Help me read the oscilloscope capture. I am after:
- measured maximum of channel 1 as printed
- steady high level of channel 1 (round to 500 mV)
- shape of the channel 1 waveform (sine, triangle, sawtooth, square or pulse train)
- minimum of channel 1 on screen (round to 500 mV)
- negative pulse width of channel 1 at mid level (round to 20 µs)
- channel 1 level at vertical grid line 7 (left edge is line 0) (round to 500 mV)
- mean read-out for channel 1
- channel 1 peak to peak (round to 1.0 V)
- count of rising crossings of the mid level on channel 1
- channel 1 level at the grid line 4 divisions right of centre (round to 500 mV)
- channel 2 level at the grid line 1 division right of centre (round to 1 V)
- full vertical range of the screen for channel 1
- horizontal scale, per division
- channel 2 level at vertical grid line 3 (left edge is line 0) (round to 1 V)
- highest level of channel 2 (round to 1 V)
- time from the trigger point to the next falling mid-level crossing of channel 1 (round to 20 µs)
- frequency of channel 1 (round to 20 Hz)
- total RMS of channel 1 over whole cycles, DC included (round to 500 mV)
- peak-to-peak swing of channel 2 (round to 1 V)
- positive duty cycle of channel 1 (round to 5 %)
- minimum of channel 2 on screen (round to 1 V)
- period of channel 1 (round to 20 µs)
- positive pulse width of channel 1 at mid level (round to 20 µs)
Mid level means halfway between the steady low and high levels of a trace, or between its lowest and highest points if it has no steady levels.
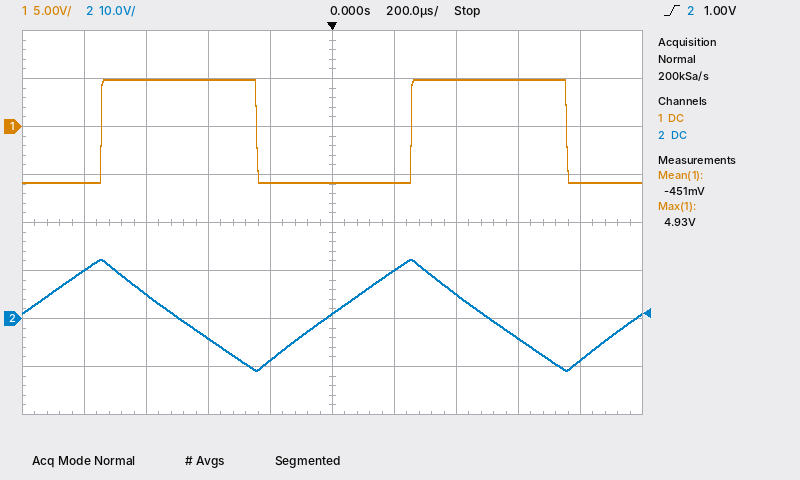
4.93 V
5.0 V
square
-6.0 V
500 µs
5.0 V
-451 mV
11.0 V
2
-6.0 V
10 V
40 V
200 µs
-4 V
12 V
760 µs
1.00 kHz
5.5 V
23 V
50 %
-11 V
1.00 ms
500 µs
